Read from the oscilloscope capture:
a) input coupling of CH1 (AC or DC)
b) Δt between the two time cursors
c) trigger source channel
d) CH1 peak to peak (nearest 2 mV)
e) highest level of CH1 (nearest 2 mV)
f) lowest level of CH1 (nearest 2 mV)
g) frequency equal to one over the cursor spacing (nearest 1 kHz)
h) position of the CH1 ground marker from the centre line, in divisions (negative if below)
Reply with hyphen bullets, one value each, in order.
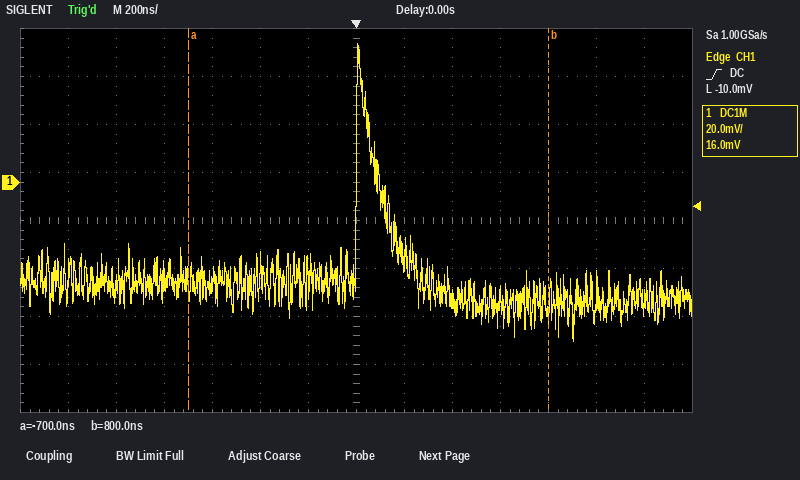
- DC
- 1.50 µs
- CH1
- 124 mV
- 58 mV
- -66 mV
- 667 kHz
- +0.8 div
